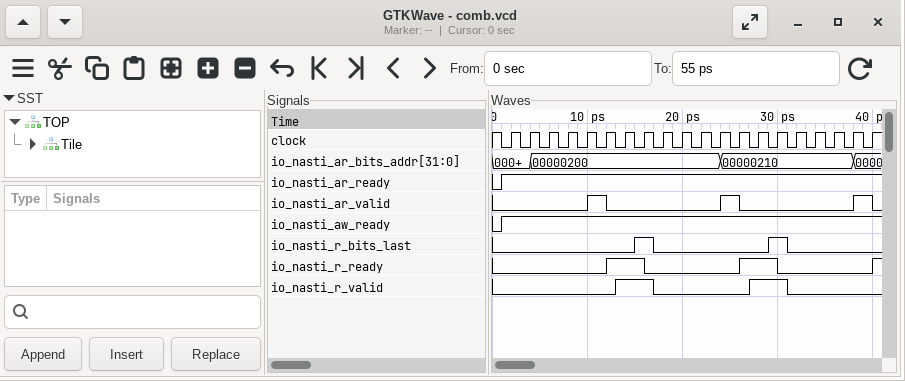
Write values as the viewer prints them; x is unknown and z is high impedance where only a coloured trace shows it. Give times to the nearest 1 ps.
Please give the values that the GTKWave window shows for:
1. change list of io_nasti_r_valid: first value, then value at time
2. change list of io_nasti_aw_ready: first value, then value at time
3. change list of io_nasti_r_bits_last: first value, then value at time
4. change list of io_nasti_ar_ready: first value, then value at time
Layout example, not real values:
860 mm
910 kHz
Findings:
0, 1 at 13 ps, 0 at 17 ps, 1 at 27 ps, 0 at 31 ps
0, 1 at 1 ps
0, 1 at 15 ps, 0 at 17 ps, 1 at 29 ps, 0 at 31 ps
0, 1 at 1 ps
